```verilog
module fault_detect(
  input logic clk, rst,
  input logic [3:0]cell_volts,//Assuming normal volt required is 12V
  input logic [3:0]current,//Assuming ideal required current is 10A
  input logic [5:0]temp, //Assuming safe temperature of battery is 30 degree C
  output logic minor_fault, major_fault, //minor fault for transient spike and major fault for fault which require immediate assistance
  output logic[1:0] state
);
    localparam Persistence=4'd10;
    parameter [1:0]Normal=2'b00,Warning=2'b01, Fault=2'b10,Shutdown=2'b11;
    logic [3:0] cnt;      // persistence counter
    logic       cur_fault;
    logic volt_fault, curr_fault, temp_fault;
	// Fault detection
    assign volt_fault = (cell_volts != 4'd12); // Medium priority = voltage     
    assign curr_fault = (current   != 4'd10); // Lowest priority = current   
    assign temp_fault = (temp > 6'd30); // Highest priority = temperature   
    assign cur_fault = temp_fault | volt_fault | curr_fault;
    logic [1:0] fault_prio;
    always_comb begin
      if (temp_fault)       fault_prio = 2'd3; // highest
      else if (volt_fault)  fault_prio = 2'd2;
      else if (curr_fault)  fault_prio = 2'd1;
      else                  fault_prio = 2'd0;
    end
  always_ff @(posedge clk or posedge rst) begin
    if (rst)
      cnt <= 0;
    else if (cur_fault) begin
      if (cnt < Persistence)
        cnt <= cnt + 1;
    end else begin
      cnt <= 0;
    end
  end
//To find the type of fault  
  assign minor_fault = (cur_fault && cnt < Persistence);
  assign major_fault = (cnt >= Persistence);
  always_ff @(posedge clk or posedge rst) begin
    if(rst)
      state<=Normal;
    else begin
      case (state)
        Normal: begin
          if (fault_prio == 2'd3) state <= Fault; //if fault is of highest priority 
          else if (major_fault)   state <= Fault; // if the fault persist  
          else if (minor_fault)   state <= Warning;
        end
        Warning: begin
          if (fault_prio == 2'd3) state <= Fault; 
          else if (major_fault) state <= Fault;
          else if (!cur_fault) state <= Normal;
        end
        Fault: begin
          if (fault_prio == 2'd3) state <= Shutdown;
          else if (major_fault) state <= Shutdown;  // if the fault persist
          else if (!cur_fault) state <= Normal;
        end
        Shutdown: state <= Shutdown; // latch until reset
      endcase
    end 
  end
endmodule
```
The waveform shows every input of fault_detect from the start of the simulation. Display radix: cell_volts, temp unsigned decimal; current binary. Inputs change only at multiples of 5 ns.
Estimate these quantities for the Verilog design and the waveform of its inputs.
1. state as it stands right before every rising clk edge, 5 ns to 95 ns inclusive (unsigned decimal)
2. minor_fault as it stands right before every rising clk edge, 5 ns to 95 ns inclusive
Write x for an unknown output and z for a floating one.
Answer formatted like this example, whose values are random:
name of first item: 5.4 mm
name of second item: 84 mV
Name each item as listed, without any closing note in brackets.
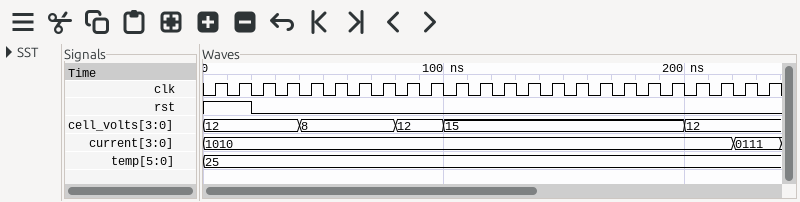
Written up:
state as it stands right before every rising clk edge, 5 ns to 95 ns inclusive: 0, 0, 0, 0, 0, 1, 1, 1, 1, 0
minor_fault as it stands right before every rising clk edge, 5 ns to 95 ns inclusive: 0 0 0 0 1 1 1 1 0 0
